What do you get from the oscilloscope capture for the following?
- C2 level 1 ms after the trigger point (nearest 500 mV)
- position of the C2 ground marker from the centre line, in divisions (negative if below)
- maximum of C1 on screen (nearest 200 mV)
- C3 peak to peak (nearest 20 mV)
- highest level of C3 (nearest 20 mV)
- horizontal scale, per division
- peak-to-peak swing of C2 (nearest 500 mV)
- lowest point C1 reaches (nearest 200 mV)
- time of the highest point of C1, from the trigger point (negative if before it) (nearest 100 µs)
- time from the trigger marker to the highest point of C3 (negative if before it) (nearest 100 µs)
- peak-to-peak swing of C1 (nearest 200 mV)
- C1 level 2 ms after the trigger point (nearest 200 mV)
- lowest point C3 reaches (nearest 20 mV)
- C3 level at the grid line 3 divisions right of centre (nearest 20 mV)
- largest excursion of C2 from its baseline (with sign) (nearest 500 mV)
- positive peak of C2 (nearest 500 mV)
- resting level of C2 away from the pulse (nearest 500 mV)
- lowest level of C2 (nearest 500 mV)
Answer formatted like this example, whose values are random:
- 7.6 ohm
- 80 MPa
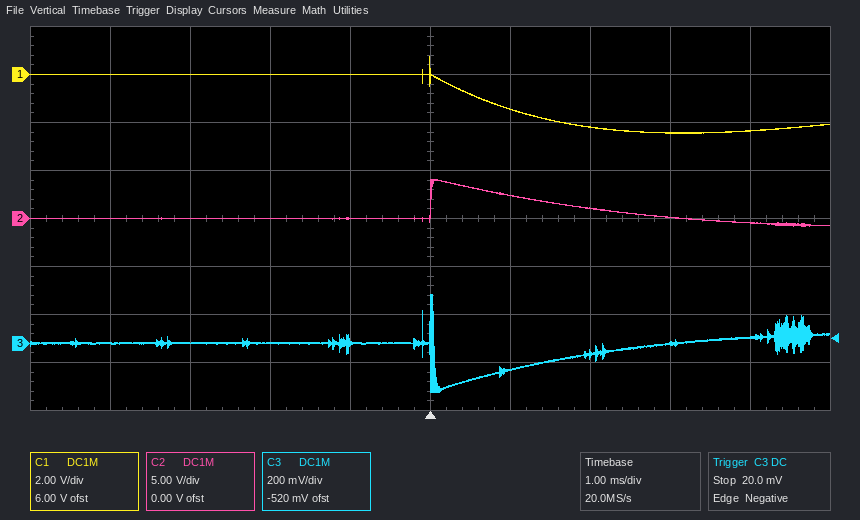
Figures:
- 2.5 V
- 0.0 div
- 800 mV
- 400 mV
- 200 mV
- 1 ms
- 5.0 V
- -2.4 V
- 0.0 ms
- 0.0 ms
- 3.2 V
- -2.2 V
- -200 mV
- 0 mV
- +4.0 V
- 4.0 V
- 0.0 V
- -1.0 V
